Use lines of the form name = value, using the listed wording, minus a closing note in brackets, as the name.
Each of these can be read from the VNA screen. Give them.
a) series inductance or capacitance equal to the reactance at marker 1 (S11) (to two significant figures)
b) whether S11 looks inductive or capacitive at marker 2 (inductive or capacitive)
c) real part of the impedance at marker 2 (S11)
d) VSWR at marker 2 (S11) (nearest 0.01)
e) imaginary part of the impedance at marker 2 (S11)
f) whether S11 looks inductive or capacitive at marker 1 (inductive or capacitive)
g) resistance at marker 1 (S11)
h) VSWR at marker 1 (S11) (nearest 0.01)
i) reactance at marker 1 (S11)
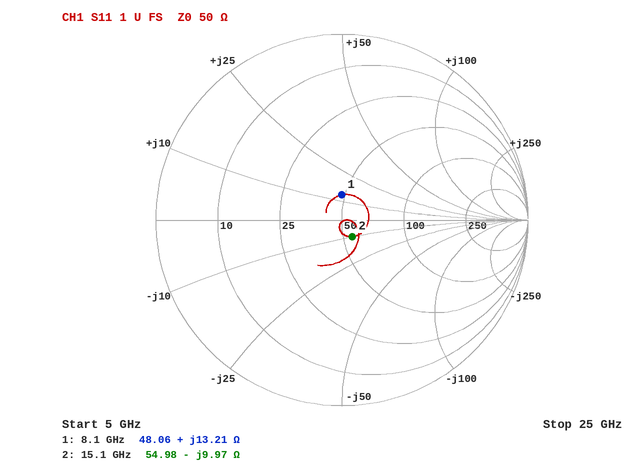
series inductance or capacitance equal to the reactance at marker 1 (S11) = 260 pH
whether S11 looks inductive or capacitive at marker 2 = capacitive
real part of the impedance at marker 2 = 54.98 Ω
VSWR at marker 2 (S11) = 1.24
imaginary part of the impedance at marker 2 = -9.97 Ω
whether S11 looks inductive or capacitive at marker 1 = inductive
resistance at marker 1 = 48.06 Ω
VSWR at marker 1 (S11) = 1.31
reactance at marker 1 = +13.21 Ω
